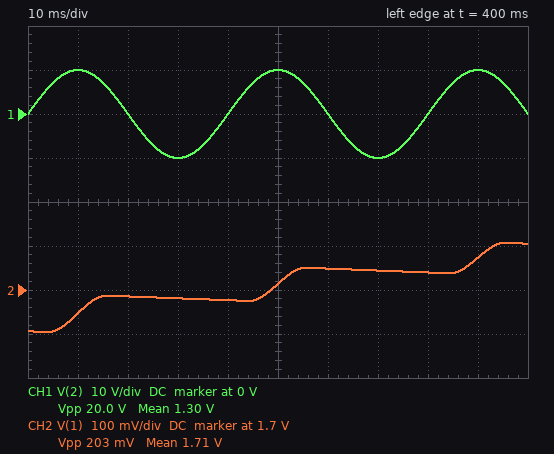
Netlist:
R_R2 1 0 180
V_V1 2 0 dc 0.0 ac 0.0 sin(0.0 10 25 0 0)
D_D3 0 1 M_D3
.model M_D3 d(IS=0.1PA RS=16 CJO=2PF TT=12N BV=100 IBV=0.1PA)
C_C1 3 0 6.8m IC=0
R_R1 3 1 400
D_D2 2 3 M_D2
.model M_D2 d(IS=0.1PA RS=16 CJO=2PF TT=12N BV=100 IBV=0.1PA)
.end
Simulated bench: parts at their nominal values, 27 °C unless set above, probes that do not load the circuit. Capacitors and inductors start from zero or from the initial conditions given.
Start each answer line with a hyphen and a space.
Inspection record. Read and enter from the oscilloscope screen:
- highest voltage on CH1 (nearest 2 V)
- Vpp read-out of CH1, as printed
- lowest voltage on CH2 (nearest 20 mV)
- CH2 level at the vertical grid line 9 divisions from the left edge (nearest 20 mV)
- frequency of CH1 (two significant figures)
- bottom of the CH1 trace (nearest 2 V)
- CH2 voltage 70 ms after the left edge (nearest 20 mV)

- 10 V
- 20.0 V
- 1.60 V
- 1.78 V
- 25 Hz
- -10 V
- 1.74 V
